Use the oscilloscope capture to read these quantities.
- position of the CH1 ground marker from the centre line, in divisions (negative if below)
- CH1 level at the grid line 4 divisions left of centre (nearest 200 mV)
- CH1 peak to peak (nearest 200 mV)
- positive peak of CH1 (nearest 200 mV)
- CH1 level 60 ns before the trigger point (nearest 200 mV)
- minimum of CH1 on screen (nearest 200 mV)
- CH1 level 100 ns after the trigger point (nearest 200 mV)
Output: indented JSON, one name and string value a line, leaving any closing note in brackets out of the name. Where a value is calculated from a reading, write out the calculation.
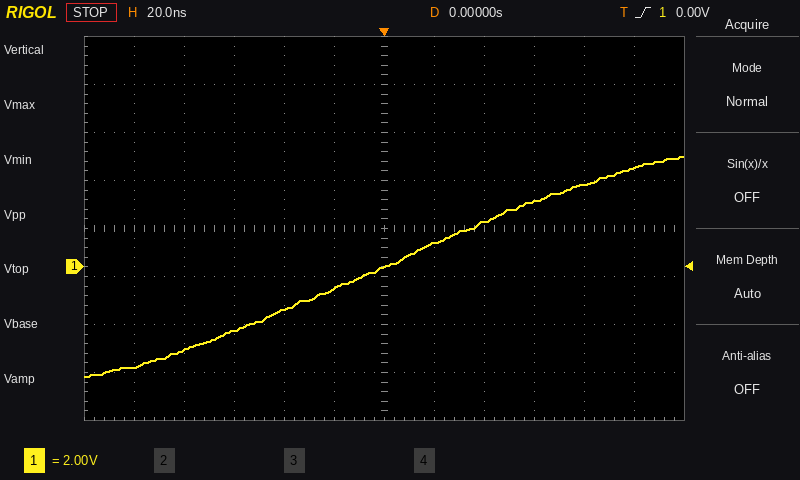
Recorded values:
{
  "position of the CH1 ground marker from the centre line, in divisions": "-0.8 div",
  "CH1 level at the grid line 4 divisions left of centre": "-3.4 V",
  "CH1 peak to peak": "4.6 V − (-4.6 V) = 9.2 V",
  "positive peak of CH1": "4.6 V",
  "CH1 level 60 ns before the trigger point": "-2.6 V",
  "minimum of CH1 on screen": "-4.6 V",
  "CH1 level 100 ns after the trigger point": "4.2 V"
}
